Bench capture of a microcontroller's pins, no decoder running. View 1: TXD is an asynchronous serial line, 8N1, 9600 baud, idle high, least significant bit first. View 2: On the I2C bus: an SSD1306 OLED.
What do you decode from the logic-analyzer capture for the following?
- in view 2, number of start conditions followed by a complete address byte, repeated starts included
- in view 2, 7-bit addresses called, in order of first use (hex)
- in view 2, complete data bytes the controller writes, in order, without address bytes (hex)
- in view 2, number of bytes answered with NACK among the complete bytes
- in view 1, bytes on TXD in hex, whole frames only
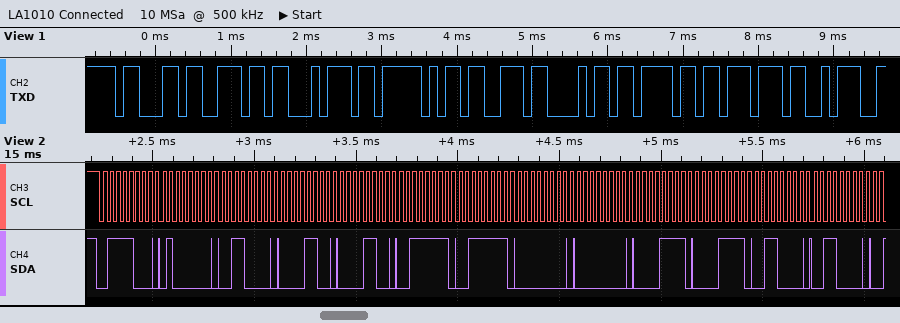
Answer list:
1
0x3C
40 30 0C 0C 3F 3F 00 00 0F 0F 30 30
0
63 6E 74 5F 73 68 6F 77 3A
